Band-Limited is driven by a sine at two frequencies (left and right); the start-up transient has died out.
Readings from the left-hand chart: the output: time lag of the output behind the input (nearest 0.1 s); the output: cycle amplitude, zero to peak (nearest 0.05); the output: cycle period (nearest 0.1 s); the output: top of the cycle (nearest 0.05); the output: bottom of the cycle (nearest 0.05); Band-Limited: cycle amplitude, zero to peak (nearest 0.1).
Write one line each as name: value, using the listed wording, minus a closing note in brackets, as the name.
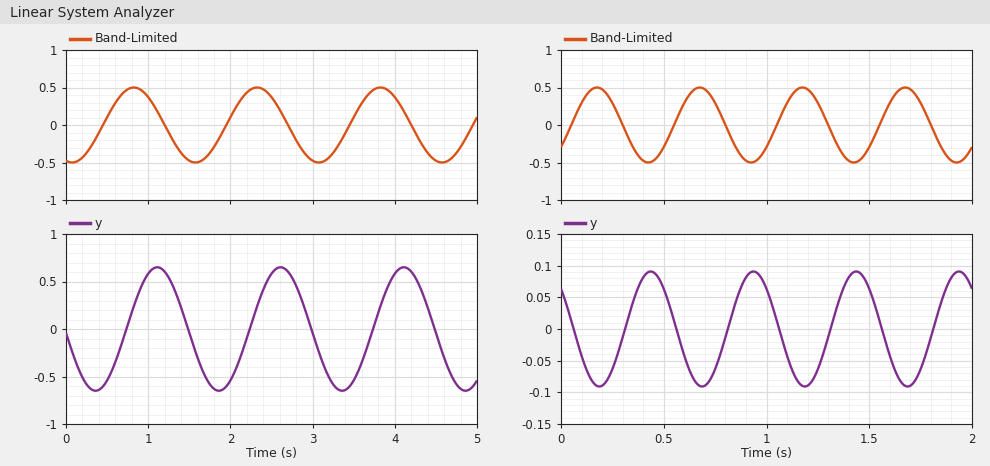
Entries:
the output: time lag of the output behind the input: 0.3 s
the output: cycle amplitude, zero to peak: 0.65
the output: cycle period: 1.5 s
the output: top of the cycle: 0.65
the output: bottom of the cycle: -0.65
Band-Limited: cycle amplitude, zero to peak: 0.5
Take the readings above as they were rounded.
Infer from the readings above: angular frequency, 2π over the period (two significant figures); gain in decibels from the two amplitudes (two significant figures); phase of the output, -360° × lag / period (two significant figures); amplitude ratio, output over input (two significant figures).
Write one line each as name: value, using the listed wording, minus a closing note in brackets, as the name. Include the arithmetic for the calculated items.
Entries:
angular frequency, 2π over the period: 2π / 1.5 = 4.2 rad/s
gain in decibels from the two amplitudes: 20 log10(0.65 / 0.5) = 2.3 dB
phase of the output, -360° × lag / period: -360 × 0.3 / 1.5 = -72°
amplitude ratio, output over input: 0.65 / 0.5 = 1.3
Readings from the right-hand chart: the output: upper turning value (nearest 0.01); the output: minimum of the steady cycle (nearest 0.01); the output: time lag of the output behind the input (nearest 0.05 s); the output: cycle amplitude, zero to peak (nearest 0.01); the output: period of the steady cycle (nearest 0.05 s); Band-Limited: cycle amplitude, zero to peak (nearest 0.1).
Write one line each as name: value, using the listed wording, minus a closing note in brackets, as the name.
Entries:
the output: upper turning value: 0.09
the output: minimum of the steady cycle: -0.09
the output: time lag of the output behind the input: 0.25 s
the output: cycle amplitude, zero to peak: 0.09
the output: period of the steady cycle: 0.50 s
Band-Limited: cycle amplitude, zero to peak: 0.5
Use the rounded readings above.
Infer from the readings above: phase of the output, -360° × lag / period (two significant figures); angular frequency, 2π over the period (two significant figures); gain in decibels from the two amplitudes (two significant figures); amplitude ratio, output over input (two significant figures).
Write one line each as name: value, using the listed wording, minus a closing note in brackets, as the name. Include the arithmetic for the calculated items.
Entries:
phase of the output, -360° × lag / period: -360 × 0.25 / 0.5 = -180°
angular frequency, 2π over the period: 2π / 0.5 = 13 rad/s
gain in decibels from the two amplitudes: 20 log10(0.09 / 0.5) = -15 dB
amplitude ratio, output over input: 0.09 / 0.5 = 0.18
